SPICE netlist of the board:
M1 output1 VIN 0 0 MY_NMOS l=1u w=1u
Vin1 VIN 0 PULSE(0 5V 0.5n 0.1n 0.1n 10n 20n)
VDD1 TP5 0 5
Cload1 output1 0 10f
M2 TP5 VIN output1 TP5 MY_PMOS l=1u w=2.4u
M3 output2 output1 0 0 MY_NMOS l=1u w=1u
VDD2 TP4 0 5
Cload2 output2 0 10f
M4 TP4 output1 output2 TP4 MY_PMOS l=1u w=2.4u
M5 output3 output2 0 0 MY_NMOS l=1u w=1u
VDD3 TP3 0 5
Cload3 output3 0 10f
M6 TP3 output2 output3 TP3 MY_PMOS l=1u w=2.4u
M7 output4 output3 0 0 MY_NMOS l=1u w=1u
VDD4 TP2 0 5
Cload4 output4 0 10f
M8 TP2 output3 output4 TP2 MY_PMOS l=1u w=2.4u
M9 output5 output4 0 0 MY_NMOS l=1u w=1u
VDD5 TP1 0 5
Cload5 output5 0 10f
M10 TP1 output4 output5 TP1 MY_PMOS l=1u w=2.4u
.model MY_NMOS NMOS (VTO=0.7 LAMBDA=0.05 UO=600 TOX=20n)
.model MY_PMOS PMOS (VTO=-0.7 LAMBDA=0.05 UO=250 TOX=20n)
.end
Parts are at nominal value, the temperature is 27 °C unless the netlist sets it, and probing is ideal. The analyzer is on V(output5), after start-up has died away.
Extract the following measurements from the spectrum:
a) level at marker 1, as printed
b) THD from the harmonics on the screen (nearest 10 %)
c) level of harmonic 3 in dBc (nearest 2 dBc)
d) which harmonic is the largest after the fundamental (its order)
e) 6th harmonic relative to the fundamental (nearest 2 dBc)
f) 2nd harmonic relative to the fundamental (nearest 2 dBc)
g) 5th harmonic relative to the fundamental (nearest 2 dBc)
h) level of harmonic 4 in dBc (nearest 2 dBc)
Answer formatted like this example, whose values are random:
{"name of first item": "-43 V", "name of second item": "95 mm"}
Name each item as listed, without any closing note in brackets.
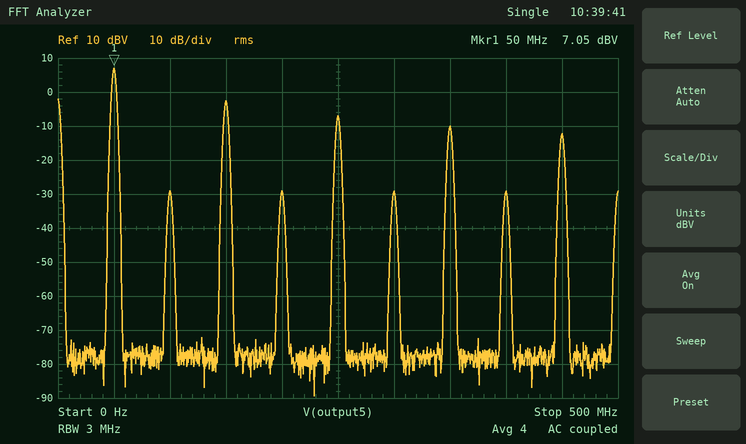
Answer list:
{"level at marker 1, as printed": "7.05 dBV", "THD from the harmonics on the screen": "40 %", "level of harmonic 3 in dBc": "-10 dBc", "which harmonic is the largest after the fundamental": "3", "6th harmonic relative to the fundamental": "-36 dBc", "2nd harmonic relative to the fundamental": "-36 dBc", "5th harmonic relative to the fundamental": "-14 dBc", "level of harmonic 4 in dBc": "-36 dBc"}
